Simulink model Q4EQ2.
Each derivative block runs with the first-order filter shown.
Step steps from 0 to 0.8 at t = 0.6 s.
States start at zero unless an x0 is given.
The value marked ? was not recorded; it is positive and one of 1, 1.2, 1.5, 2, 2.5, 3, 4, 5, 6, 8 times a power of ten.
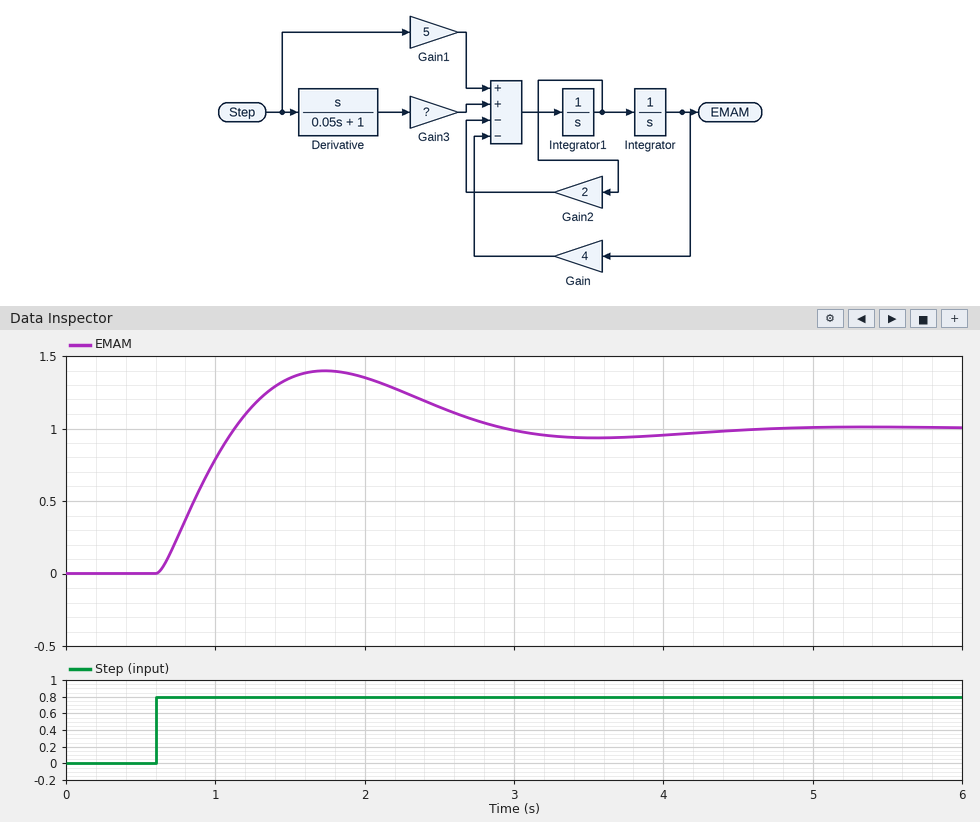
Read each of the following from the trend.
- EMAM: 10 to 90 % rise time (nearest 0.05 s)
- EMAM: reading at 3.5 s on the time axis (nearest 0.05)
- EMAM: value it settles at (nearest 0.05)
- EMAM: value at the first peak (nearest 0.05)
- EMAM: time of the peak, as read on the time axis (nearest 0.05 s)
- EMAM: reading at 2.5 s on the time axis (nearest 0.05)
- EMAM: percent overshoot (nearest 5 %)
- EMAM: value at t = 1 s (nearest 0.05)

0.40 s
0.95
1.00
1.40
1.75 s
1.15
40 %
0.80
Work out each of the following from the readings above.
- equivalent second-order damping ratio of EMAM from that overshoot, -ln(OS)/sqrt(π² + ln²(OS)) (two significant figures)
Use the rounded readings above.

0.28
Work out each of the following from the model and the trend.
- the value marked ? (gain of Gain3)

3
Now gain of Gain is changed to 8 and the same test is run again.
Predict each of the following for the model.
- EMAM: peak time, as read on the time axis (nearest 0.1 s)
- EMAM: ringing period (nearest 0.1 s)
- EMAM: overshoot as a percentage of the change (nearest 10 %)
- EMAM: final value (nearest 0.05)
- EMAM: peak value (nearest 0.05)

1.3 s
2.4 s
90 %
0.50
0.95
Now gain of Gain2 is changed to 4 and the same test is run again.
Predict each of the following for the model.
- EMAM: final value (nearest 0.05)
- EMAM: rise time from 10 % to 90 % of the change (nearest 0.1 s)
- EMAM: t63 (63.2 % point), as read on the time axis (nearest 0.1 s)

1.00
0.8 s
1.0 s
